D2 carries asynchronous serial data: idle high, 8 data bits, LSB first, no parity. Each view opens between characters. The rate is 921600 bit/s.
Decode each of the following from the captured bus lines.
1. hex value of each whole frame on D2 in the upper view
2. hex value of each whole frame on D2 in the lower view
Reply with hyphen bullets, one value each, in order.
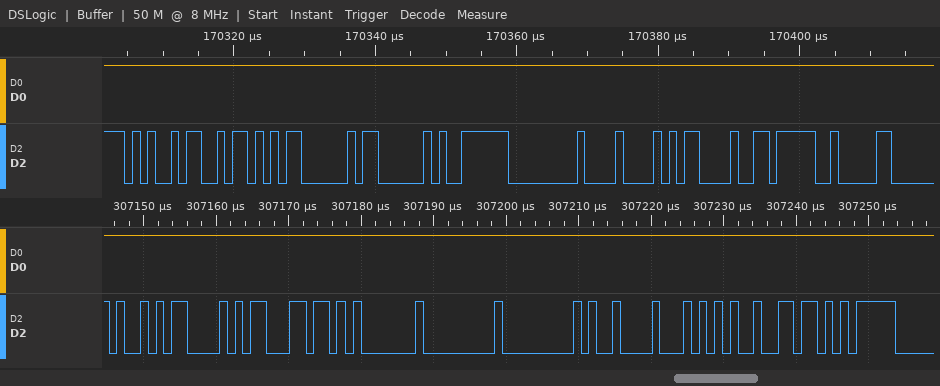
- A5, 5A, 03, 03, F9, 00, 08, 0D, F6, 82
- A9, A8, 6C, 01, 00, 00, 09, 54, B2, F5
